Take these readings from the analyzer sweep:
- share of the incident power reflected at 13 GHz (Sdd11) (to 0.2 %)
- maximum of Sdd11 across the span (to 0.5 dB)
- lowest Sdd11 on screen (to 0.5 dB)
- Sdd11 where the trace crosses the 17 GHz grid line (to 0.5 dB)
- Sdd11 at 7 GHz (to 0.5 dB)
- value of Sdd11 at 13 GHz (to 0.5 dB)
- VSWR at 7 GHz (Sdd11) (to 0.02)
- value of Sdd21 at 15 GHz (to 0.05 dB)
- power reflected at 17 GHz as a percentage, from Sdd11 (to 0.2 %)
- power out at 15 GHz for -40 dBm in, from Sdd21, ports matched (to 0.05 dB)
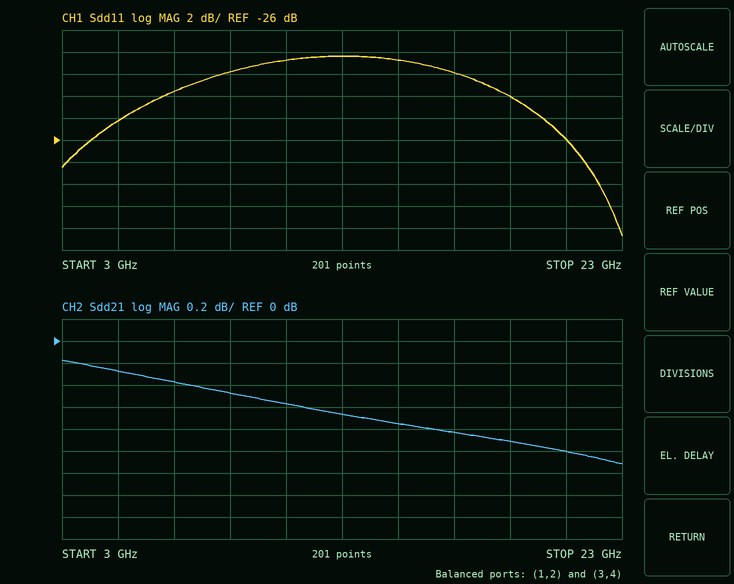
1.4 %
-18.5 dB
-34.5 dB
-20.0 dB
-21.5 dB
-18.5 dB
1.18
-0.75 dB
1.0 %
-40.75 dBm
